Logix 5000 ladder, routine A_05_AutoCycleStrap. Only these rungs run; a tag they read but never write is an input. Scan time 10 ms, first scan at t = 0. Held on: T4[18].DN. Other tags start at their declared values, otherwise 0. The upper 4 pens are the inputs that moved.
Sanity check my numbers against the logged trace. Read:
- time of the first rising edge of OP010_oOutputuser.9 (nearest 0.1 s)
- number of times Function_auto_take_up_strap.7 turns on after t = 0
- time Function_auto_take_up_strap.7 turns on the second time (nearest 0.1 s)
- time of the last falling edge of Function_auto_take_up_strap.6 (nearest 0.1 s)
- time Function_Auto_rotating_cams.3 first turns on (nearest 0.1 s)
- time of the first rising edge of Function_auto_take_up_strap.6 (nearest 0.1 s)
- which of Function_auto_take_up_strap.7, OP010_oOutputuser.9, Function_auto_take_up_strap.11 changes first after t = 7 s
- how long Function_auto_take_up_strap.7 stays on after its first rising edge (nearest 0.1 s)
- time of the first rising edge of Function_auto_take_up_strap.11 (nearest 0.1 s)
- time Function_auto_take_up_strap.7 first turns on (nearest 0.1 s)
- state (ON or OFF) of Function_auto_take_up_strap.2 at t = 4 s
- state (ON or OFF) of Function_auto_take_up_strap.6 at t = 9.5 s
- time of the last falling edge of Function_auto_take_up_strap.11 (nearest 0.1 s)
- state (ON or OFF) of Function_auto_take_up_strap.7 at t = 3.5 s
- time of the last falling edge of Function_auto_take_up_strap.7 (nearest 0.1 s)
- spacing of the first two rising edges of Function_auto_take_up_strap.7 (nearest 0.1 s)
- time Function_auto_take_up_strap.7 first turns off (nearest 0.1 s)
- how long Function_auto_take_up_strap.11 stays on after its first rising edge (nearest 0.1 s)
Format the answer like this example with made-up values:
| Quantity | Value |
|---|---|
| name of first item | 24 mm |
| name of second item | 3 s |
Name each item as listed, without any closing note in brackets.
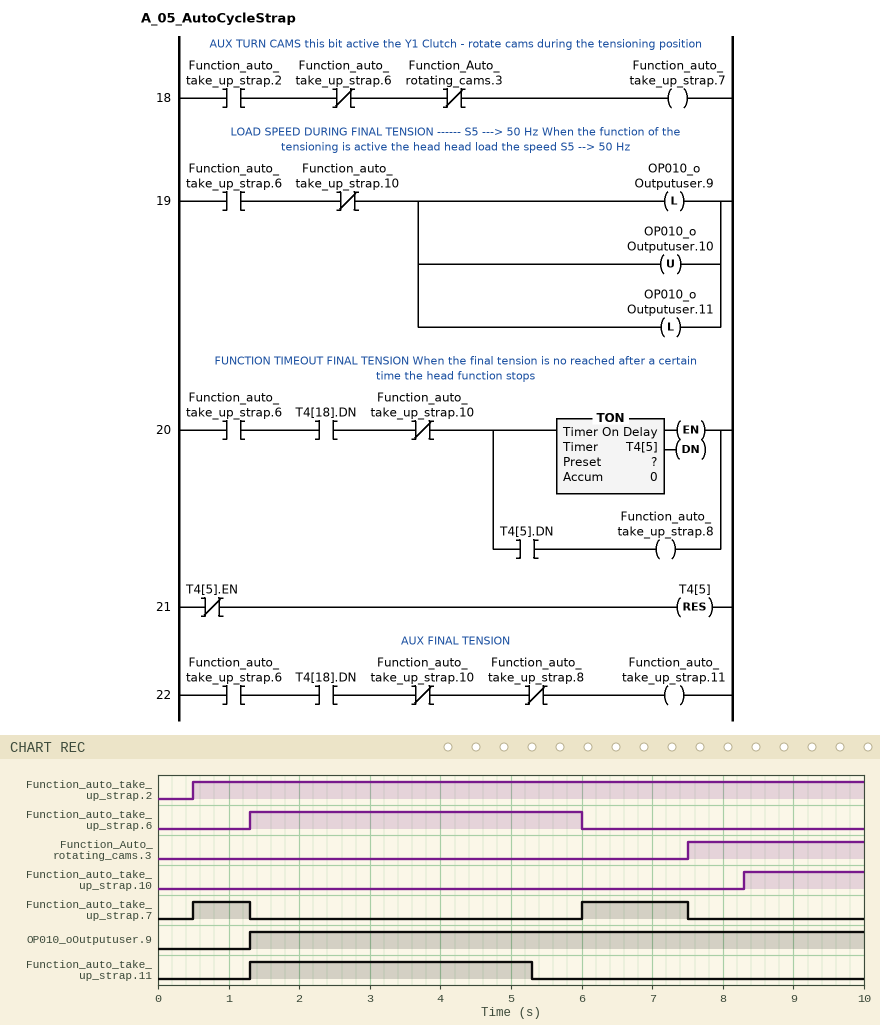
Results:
| Quantity | Value |
|---|---|
| time of the first rising edge of OP010_oOutputuser.9 | 1.3 s |
| number of times Function_auto_take_up_strap.7 turns on after t = 0 | 2 |
| time Function_auto_take_up_strap.7 turns on the second time | 6.0 s |
| time of the last falling edge of Function_auto_take_up_strap.6 | 6.0 s |
| time Function_Auto_rotating_cams.3 first turns on | 7.5 s |
| time of the first rising edge of Function_auto_take_up_strap.6 | 1.3 s |
| which of Function_auto_take_up_strap.7, OP010_oOutputuser.9, Function_auto_take_up_strap.11 changes first after t = 7 s | Function_auto_take_up_strap.7 |
| how long Function_auto_take_up_strap.7 stays on after its first rising edge | 0.8 s |
| time of the first rising edge of Function_auto_take_up_strap.11 | 1.3 s |
| time Function_auto_take_up_strap.7 first turns on | 0.5 s |
| state (ON or OFF) of Function_auto_take_up_strap.2 at t = 4 s | ON |
| state (ON or OFF) of Function_auto_take_up_strap.6 at t = 9.5 s | OFF |
| time of the last falling edge of Function_auto_take_up_strap.11 | 5.3 s |
| state (ON or OFF) of Function_auto_take_up_strap.7 at t = 3.5 s | OFF |
| time of the last falling edge of Function_auto_take_up_strap.7 | 7.5 s |
| spacing of the first two rising edges of Function_auto_take_up_strap.7 | 5.5 s |
| time Function_auto_take_up_strap.7 first turns off | 1.3 s |
| how long Function_auto_take_up_strap.11 stays on after its first rising edge | 4.0 s |
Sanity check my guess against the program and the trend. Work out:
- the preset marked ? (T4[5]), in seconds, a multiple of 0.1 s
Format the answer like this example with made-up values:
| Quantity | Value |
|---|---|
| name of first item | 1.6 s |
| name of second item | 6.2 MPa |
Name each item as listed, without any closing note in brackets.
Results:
| Quantity | Value |
|---|---|
| the preset marked ? (T4[5]), in seconds, a multiple of 0.1 s | 4.0 s |
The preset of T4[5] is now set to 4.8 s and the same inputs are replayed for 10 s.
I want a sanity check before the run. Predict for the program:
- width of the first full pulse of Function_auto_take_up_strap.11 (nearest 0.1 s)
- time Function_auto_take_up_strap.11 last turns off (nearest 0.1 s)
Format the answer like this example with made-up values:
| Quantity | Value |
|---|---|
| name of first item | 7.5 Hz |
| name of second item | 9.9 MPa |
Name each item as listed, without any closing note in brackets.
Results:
| Quantity | Value |
|---|---|
| width of the first full pulse of Function_auto_take_up_strap.11 | 4.7 s |
| time Function_auto_take_up_strap.11 last turns off | 6.0 s |
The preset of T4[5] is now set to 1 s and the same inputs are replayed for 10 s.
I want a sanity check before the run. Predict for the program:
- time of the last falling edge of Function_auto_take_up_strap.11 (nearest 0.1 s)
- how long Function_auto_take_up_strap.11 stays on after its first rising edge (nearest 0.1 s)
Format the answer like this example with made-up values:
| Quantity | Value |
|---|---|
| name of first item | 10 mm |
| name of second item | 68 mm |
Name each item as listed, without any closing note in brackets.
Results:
| Quantity | Value |
|---|---|
| time of the last falling edge of Function_auto_take_up_strap.11 | 2.3 s |
| how long Function_auto_take_up_strap.11 stays on after its first rising edge | 1.0 s |
